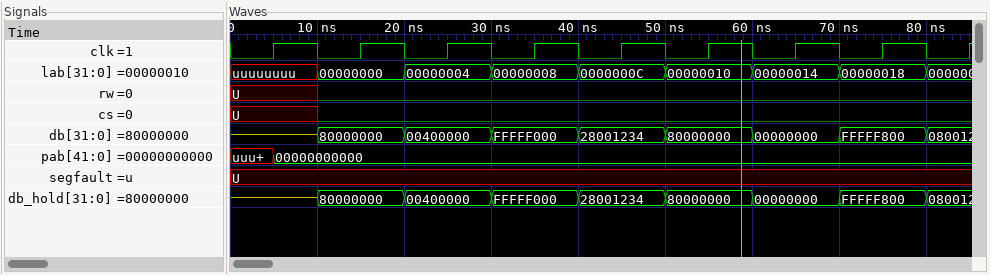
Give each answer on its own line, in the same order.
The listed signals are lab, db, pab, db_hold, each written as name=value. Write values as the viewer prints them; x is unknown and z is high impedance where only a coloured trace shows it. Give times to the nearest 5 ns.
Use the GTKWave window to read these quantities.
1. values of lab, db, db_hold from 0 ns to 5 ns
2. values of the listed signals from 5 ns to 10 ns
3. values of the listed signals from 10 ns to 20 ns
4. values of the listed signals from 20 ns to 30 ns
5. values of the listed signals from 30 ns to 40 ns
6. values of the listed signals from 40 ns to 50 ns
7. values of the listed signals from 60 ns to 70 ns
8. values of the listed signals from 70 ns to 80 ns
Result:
lab=uuuuuuuu, db=z, db_hold=z
lab=uuuuuuuu, db=z, pab=00000000000, db_hold=z
lab=00000000, db=80000000, pab=00000000000, db_hold=80000000
lab=00000004, db=00400000, pab=00000000000, db_hold=00400000
lab=00000008, db=FFFFF000, pab=00000000000, db_hold=FFFFF000
lab=0000000C, db=28001234, pab=00000000000, db_hold=28001234
lab=00000014, db=00000000, pab=00000000000, db_hold=00000000
lab=00000018, db=FFFFF800, pab=00000000000, db_hold=FFFFF800
